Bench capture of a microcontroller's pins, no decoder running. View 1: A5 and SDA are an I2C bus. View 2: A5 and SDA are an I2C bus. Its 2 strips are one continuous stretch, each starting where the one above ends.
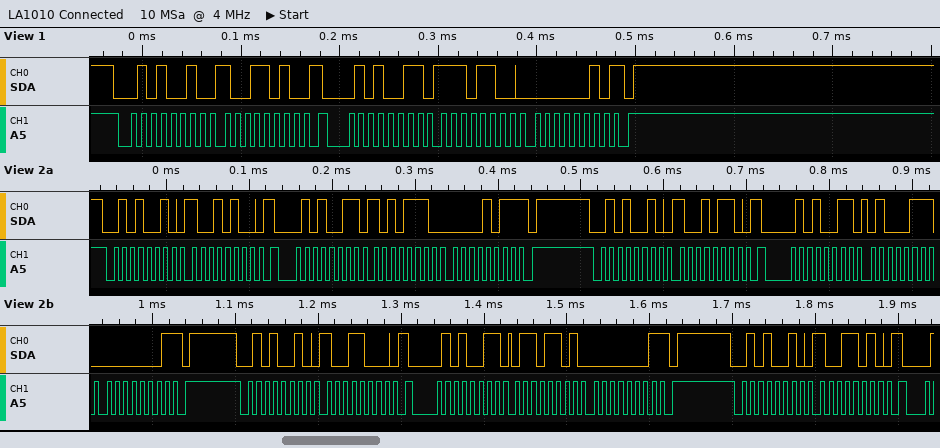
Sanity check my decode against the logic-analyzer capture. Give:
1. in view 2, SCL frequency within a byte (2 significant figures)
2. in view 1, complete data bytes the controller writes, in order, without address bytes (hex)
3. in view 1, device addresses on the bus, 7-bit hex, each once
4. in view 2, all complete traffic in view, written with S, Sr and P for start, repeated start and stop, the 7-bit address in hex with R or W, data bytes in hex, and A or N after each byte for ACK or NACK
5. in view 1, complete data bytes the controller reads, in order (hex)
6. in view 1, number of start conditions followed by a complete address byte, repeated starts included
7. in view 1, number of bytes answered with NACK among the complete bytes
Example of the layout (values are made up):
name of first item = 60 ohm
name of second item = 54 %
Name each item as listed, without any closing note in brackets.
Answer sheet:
in view 2, SCL frequency within a byte = 100 kHz
in view 1, complete data bytes the controller writes, in order, without address bytes = 9A
in view 1, device addresses on the bus, 7-bit hex, each once = 0x29
in view 2, all complete traffic in view, written with S, Sr and P for start, repeated start and stop, the 7-bit address in hex with R or W, data bytes in hex, and A or N after each byte for ACK or NACK = S 29W A 94 A Sr 29R A AE A 0B N P S 29W A 96 A Sr 29R A 47 A 01 N P S 29W A 98 A Sr 29R A 6D A 01 N P S 29W A 9A A
in view 1, complete data bytes the controller reads, in order = EC 02
in view 1, number of start conditions followed by a complete address byte, repeated starts included = 2
in view 1, number of bytes answered with NACK among the complete bytes = 1
